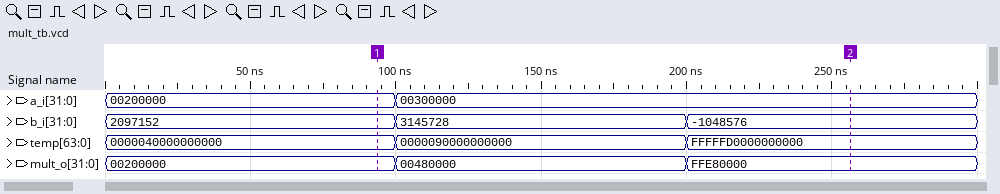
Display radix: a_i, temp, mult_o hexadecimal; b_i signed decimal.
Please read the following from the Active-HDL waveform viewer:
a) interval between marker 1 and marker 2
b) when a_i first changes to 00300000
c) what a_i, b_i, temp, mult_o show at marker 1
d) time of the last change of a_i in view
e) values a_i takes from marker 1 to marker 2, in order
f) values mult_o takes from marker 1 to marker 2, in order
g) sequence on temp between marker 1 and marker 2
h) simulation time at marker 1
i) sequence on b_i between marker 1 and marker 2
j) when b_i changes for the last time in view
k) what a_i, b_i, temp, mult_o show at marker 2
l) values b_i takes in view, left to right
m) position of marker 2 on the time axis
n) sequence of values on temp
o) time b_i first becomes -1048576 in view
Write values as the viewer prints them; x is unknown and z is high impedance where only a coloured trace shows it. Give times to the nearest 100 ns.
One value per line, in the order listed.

200 ns
100 ns
a_i=00200000, b_i=2097152, temp=0000040000000000, mult_o=00200000
100 ns
00200000, 00300000
00200000, 00480000, FFE80000
0000040000000000, 0000090000000000, FFFFFD0000000000
100 ns
2097152, 3145728, -1048576
200 ns
a_i=00300000, b_i=-1048576, temp=FFFFFD0000000000, mult_o=FFE80000
2097152, 3145728, -1048576
300 ns
0000040000000000, 0000090000000000, FFFFFD0000000000
200 ns
